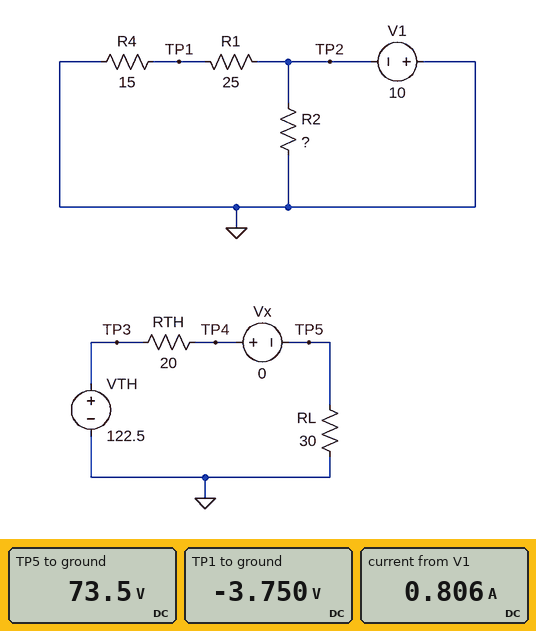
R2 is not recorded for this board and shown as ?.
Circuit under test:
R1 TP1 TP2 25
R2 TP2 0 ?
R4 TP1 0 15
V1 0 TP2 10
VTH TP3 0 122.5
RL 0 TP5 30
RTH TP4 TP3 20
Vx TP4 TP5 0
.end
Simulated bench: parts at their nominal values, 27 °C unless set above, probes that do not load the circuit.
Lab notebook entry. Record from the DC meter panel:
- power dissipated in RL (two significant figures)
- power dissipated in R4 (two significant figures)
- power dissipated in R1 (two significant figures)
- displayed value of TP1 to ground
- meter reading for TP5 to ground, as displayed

180 W
940 mW
1.6 W
-3.750 V
73.5 V
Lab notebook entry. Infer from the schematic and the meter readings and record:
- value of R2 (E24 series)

18 Ω
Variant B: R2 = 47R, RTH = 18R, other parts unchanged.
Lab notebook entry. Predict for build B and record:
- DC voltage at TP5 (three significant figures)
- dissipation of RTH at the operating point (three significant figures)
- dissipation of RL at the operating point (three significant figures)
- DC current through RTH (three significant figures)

76.6 V
117 W
195 W
2.55 A
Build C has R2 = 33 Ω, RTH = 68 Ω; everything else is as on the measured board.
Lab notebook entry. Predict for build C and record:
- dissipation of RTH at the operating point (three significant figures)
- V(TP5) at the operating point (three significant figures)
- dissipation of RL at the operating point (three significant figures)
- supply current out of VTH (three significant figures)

106 W
37.5 V
46.9 W
1.25 A
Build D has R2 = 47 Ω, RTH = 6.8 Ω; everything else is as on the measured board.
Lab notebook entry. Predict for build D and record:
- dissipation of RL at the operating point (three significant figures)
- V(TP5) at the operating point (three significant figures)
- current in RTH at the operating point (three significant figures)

332 W
99.9 V
3.33 A
